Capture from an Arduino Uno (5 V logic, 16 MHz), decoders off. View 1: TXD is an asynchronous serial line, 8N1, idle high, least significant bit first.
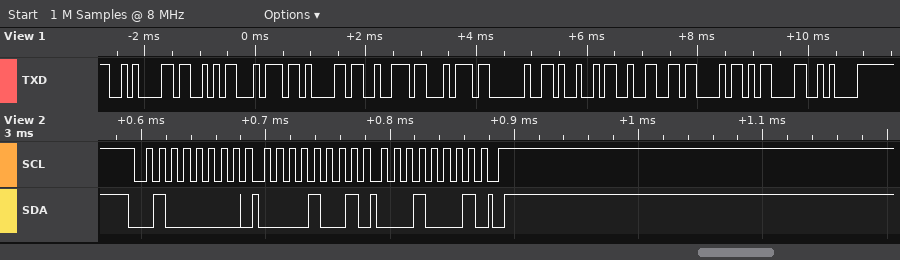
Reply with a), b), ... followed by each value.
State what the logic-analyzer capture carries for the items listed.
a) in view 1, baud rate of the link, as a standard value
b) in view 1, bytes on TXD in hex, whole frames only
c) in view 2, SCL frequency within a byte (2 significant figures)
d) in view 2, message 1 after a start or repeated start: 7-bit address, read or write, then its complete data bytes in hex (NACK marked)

a) 9600 baud
b) 0A 53 74 61 72 74 20 49 32 43 0D 0A
c) 100 kHz
d) 0x20 write: 09 11
